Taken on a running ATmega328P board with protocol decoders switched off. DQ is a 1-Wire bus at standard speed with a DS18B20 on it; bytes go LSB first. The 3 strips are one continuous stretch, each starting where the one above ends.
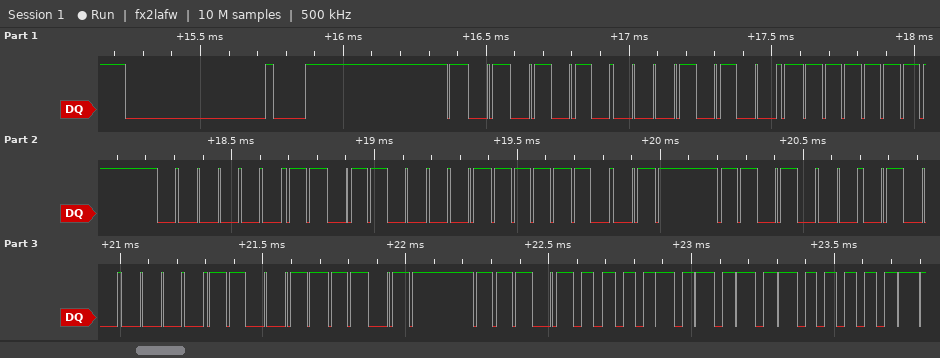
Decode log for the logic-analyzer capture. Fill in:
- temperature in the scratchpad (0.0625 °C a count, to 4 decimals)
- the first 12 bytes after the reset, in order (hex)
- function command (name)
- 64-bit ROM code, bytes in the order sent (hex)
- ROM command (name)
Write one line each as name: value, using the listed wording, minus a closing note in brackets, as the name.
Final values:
temperature in the scratchpad: 85.0000 °C
the first 12 bytes after the reset, in order: 55 28 FF C0 86 9F 17 02 F3 BE 50 05
function command: Read Scratchpad
64-bit ROM code, bytes in the order sent: 28 FF C0 86 9F 17 02 F3
ROM command: Match ROM
